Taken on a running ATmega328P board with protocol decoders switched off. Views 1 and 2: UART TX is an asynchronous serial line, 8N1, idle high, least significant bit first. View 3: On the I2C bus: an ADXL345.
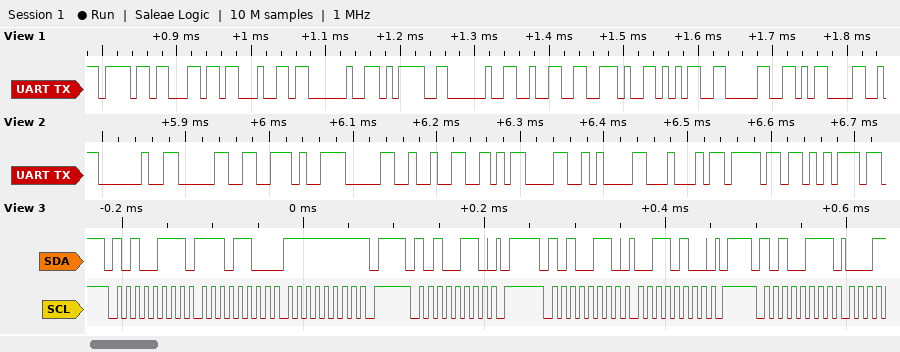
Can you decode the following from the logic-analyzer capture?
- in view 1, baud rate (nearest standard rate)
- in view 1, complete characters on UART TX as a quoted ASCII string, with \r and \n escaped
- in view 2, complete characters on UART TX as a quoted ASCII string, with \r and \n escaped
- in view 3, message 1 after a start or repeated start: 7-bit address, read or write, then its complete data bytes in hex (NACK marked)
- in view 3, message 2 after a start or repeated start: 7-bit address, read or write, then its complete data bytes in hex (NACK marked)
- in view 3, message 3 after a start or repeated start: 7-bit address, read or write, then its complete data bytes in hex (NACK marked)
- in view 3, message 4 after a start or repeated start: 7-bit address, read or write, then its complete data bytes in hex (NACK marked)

115200 baud
"old = 2.50\r"
" 0.02\r\nDou"
0x53 read: EC FF NACK
0x53 write
0x53 write: 34
0x53 read
